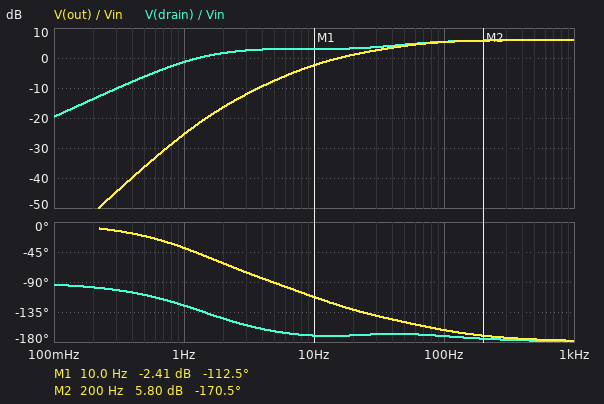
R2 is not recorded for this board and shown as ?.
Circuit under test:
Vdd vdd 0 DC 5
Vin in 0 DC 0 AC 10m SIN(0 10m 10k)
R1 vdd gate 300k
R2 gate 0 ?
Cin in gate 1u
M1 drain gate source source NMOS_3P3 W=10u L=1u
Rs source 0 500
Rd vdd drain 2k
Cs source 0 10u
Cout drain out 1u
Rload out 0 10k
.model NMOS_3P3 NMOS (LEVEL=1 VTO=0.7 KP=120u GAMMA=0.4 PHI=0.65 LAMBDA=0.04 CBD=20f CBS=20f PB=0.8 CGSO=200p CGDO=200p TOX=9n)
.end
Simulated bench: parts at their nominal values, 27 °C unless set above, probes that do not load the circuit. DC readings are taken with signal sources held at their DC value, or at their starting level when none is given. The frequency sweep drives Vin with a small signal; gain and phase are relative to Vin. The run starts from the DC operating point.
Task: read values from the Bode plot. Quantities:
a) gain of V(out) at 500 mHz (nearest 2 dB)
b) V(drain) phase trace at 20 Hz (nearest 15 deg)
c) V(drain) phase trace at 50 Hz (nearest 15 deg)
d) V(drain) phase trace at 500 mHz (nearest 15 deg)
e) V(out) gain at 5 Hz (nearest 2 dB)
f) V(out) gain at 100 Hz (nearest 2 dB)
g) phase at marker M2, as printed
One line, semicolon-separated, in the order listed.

-36 dB; -165 deg; -165 deg; -105 deg; -8 dB; 6 dB; -170.5 deg
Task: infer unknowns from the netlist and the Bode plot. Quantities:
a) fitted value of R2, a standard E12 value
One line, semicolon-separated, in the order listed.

180 kΩ
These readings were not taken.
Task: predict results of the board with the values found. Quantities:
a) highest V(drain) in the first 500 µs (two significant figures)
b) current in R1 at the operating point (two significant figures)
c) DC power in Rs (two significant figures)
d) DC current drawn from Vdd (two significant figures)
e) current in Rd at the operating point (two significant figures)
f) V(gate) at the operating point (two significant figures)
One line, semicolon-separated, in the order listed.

3.9 V; 10 µA; 150 µW; 560 µA; 550 µA; 1.9 V
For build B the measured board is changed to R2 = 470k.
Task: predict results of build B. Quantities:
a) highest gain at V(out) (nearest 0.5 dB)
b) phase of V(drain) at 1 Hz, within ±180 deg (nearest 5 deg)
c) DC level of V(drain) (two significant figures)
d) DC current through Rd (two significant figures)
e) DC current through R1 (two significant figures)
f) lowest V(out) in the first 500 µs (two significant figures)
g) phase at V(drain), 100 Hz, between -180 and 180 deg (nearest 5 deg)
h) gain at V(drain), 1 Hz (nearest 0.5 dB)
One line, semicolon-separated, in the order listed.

2.5 dB; -140 deg; 2.0 V; 1.5 mA; 6.5 µA; -13 mV; -170 deg; -2.5 dB
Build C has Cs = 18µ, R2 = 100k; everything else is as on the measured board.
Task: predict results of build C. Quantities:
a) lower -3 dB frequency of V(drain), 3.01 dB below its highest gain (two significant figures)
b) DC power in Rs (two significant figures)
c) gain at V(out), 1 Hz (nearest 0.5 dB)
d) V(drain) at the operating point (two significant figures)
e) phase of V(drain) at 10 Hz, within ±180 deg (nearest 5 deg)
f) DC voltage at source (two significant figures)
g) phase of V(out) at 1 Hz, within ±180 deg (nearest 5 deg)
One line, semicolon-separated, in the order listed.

2.7 Hz; 12 µW; -31.5 dB; 4.7 V; -165 deg; 79 mV; -30 deg
